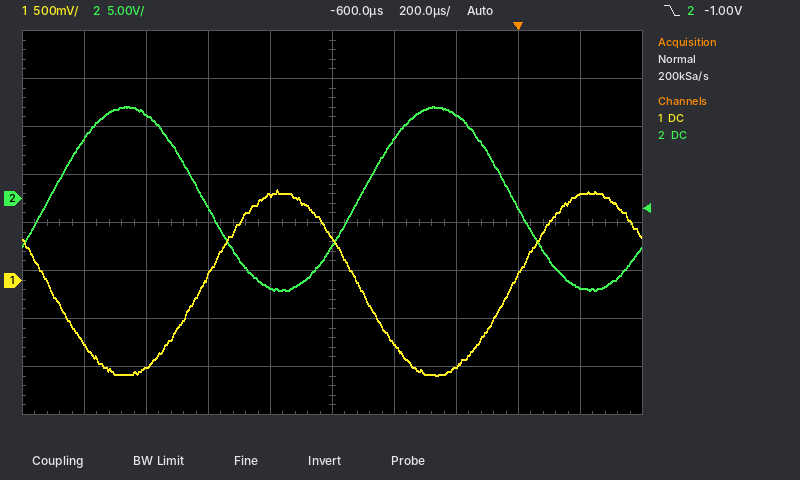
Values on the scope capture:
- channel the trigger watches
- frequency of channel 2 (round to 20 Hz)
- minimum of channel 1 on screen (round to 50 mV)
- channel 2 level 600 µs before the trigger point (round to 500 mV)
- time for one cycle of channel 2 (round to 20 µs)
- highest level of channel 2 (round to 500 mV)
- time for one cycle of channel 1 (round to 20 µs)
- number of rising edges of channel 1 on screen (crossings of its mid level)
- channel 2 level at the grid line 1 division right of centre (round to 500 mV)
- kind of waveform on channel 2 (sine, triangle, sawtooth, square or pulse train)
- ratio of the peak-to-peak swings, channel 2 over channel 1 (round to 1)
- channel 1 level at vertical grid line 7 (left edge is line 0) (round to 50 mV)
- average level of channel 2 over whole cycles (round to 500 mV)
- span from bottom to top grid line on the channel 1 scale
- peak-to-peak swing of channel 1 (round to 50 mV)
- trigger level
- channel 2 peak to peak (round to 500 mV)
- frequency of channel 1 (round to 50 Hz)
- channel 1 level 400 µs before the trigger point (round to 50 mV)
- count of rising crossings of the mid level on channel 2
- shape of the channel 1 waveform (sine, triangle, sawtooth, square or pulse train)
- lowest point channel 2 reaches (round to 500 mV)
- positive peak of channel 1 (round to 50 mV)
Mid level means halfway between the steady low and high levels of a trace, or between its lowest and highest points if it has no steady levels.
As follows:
channel 2
1.00 kHz
-1.00 V
-5.0 V
1.00 ms
9.5 V
1.00 ms
2
6.0 V
sine
10
-900 mV
0.0 V
4 V
1.95 V
-1.00 V
19.0 V
1.00 kHz
-650 mV
2
sine
-9.5 V
950 mV
